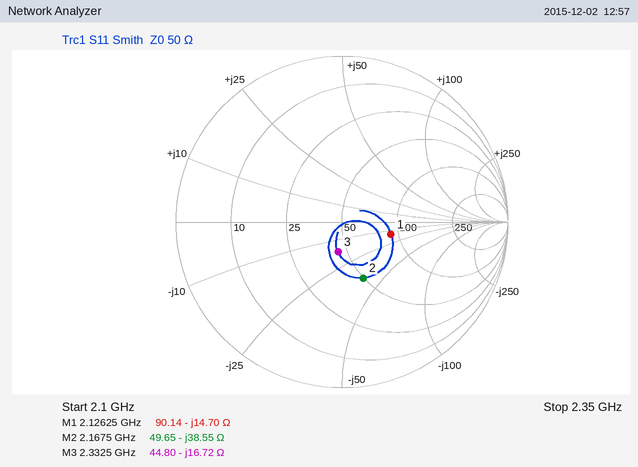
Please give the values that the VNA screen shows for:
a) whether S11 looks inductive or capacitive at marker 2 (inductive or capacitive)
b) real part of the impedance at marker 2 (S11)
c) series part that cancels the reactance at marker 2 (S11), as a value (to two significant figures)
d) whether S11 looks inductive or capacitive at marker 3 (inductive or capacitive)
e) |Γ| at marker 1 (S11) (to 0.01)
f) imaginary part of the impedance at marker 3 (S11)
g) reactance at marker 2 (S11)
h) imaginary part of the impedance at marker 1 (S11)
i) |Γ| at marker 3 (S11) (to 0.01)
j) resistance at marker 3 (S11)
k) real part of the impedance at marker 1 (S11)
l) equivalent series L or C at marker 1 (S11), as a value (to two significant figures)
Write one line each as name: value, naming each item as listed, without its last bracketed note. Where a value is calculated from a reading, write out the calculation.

whether S11 looks inductive or capacitive at marker 2: capacitive
real part of the impedance at marker 2: 49.65 Ω
series part that cancels the reactance at marker 2 (S11), as a value: L = 38.55 Ω/(2π × 2.1675 GHz) ≈ 2.8 nH
whether S11 looks inductive or capacitive at marker 3: capacitive
|Γ| at marker 1 (S11): 0.30
imaginary part of the impedance at marker 3: -16.72 Ω
reactance at marker 2: -38.55 Ω
imaginary part of the impedance at marker 1: -14.70 Ω
|Γ| at marker 3 (S11): 0.18
resistance at marker 3: 44.80 Ω
real part of the impedance at marker 1: 90.14 Ω
equivalent series L or C at marker 1 (S11), as a value: C = 1/(2π × 2.12625 GHz × 14.7 Ω) ≈ 5.1 pF
